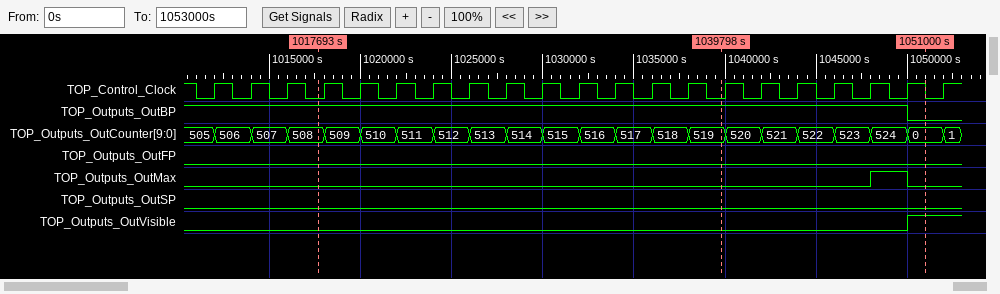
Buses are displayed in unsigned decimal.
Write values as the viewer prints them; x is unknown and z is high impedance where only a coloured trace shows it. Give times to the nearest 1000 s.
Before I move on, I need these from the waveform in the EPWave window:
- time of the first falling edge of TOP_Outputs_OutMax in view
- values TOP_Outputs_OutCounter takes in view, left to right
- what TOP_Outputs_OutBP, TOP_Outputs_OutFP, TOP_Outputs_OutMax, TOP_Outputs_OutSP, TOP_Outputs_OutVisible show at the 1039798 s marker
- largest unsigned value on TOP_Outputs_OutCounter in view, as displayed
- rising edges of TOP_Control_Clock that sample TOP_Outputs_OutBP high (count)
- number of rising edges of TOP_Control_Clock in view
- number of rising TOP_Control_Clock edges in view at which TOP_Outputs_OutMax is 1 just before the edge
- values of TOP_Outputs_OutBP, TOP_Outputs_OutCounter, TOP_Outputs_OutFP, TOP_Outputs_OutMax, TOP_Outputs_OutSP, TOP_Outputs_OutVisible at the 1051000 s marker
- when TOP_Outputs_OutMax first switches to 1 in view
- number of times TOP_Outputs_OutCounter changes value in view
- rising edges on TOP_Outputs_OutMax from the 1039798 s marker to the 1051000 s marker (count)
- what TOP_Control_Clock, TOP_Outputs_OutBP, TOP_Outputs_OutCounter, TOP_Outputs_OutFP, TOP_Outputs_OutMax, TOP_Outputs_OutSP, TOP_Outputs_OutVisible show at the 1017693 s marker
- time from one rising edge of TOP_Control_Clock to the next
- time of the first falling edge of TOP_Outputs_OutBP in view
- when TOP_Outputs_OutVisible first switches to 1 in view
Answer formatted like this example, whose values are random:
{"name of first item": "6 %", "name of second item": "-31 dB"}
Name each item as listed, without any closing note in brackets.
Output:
{"time of the first falling edge of TOP_Outputs_OutMax in view": "1050000 s", "values TOP_Outputs_OutCounter takes in view, left to right": "505, 506, 507, 508, 509, 510, 511, 512, 513, 514, 515, 516, 517, 518, 519, 520, 521, 522, 523, 524, 0, 1", "what TOP_Outputs_OutBP, TOP_Outputs_OutFP, TOP_Outputs_OutMax, TOP_Outputs_OutSP, TOP_Outputs_OutVisible show at the 1039798 s marker": "TOP_Outputs_OutBP=1, TOP_Outputs_OutFP=0, TOP_Outputs_OutMax=0, TOP_Outputs_OutSP=0, TOP_Outputs_OutVisible=0", "largest unsigned value on TOP_Outputs_OutCounter in view, as displayed": "524", "rising edges of TOP_Control_Clock that sample TOP_Outputs_OutBP high": "20", "number of rising edges of TOP_Control_Clock in view": "21", "number of rising TOP_Control_Clock edges in view at which TOP_Outputs_OutMax is 1 just before the edge": "1", "values of TOP_Outputs_OutBP, TOP_Outputs_OutCounter, TOP_Outputs_OutFP, TOP_Outputs_OutMax, TOP_Outputs_OutSP, TOP_Outputs_OutVisible at the 1051000 s marker": "TOP_Outputs_OutBP=0, TOP_Outputs_OutCounter=0, TOP_Outputs_OutFP=0, TOP_Outputs_OutMax=0, TOP_Outputs_OutSP=0, TOP_Outputs_OutVisible=1", "when TOP_Outputs_OutMax first switches to 1 in view": "1048000 s", "number of times TOP_Outputs_OutCounter changes value in view": "21", "rising edges on TOP_Outputs_OutMax from the 1039798 s marker to the 1051000 s marker": "1", "what TOP_Control_Clock, TOP_Outputs_OutBP, TOP_Outputs_OutCounter, TOP_Outputs_OutFP, TOP_Outputs_OutMax, TOP_Outputs_OutSP, TOP_Outputs_OutVisible show at the 1017693 s marker": "TOP_Control_Clock=0, TOP_Outputs_OutBP=1, TOP_Outputs_OutCounter=508, TOP_Outputs_OutFP=0, TOP_Outputs_OutMax=0, TOP_Outputs_OutSP=0, TOP_Outputs_OutVisible=0", "time from one rising edge of TOP_Control_Clock to the next": "2000 s", "time of the first falling edge of TOP_Outputs_OutBP in view": "1050000 s", "when TOP_Outputs_OutVisible first switches to 1 in view": "1050000 s"}
